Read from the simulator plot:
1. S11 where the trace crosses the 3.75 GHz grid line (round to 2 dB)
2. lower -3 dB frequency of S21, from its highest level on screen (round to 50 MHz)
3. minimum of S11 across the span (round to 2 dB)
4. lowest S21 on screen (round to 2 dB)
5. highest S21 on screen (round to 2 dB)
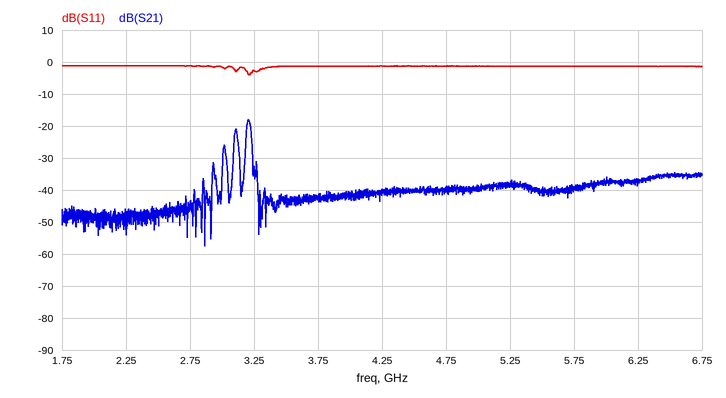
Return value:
-2 dB
3.20 GHz
-4 dB
-58 dB
-18 dB
